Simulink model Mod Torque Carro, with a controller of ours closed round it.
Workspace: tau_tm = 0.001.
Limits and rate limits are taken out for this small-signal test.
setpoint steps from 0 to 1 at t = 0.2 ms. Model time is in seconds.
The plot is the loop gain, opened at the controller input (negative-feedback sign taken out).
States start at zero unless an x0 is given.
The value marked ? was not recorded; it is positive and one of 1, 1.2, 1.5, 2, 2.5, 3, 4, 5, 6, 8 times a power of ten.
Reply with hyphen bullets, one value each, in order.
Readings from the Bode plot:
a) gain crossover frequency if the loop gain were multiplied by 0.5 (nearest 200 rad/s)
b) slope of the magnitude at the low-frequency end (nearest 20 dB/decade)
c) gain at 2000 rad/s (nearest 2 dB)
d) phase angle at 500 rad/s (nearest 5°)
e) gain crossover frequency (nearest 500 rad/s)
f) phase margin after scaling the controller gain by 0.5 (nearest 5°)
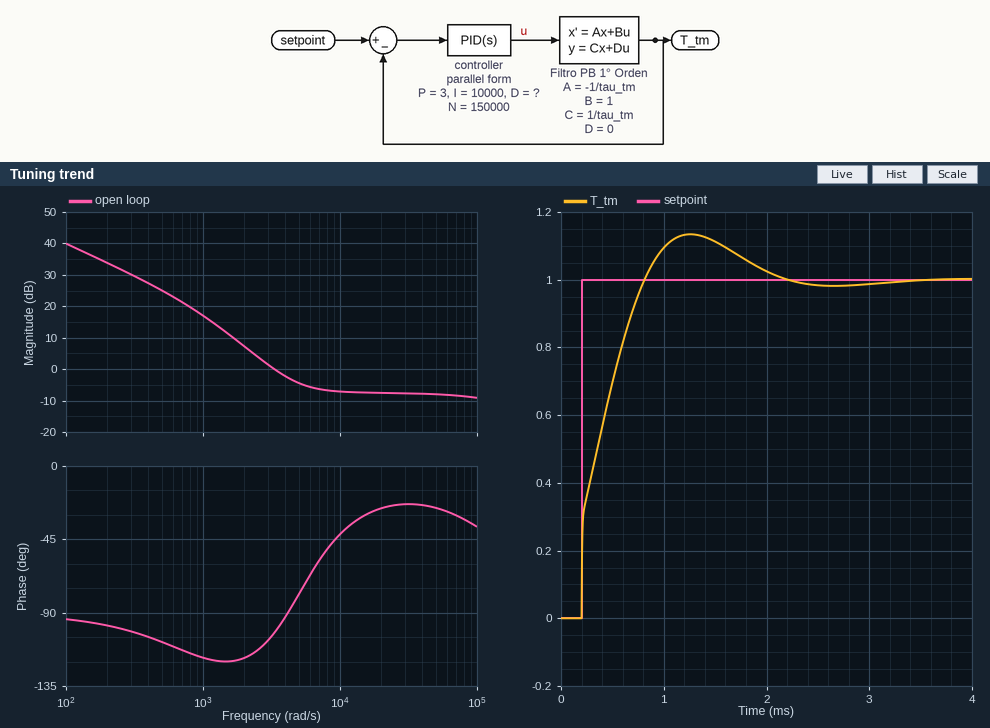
- 2200 rad/s
- -20 dB/decade
- 8 dB
- -110°
- 3500 rad/s
- 65°
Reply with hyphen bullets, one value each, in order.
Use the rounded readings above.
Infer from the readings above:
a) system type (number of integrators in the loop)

- 1
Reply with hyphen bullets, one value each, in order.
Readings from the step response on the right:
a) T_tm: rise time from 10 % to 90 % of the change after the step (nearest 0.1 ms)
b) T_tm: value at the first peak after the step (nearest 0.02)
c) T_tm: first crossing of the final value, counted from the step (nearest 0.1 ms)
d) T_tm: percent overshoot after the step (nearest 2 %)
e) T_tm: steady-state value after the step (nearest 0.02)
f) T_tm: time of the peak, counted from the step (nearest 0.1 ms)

- 0.5 ms
- 1.14
- 0.6 ms
- 14 %
- 1.00
- 1.1 ms
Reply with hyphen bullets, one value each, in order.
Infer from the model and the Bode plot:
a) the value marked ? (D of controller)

- 0.0004
